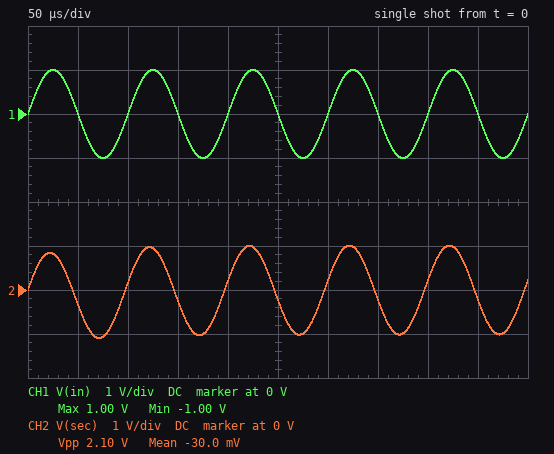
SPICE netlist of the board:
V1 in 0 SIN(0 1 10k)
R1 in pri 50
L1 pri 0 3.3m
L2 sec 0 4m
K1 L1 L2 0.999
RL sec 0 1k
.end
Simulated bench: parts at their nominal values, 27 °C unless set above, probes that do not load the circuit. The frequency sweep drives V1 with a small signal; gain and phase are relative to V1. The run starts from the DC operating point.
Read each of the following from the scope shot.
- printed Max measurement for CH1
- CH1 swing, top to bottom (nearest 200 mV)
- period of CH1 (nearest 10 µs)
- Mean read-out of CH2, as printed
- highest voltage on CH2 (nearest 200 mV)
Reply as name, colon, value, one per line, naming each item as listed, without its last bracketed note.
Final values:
printed Max measurement for CH1: 1.00 V
CH1 swing, top to bottom: 2.0 V
period of CH1: 100 µs
Mean read-out of CH2, as printed: -30.0 mV
highest voltage on CH2: 1.0 V
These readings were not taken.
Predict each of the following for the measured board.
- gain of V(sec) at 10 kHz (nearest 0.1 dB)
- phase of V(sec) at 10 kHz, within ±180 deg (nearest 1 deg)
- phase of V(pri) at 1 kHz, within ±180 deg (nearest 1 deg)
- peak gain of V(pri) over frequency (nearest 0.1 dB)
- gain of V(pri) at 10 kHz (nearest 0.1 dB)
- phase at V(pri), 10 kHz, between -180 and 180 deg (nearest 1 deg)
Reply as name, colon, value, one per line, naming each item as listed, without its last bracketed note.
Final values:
gain of V(sec) at 10 kHz: 0.1 dB
phase of V(sec) at 10 kHz, within ±180 deg: 13 deg
phase of V(pri) at 1 kHz, within ±180 deg: 66 deg
peak gain of V(pri) over frequency: 0 dB
gain of V(pri) at 10 kHz: -0.7 dB
phase at V(pri), 10 kHz, between -180 and 180 deg: 13 deg
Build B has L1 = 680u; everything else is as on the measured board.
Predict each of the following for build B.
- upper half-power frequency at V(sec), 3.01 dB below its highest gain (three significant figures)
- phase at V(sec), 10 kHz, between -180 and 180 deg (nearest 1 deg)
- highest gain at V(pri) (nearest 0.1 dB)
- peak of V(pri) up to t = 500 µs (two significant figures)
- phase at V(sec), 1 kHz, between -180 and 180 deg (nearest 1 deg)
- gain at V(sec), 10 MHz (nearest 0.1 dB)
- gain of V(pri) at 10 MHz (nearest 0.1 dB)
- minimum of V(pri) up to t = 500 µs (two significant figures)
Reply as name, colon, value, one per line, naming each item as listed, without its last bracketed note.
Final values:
upper half-power frequency at V(sec), 3.01 dB below its highest gain: 25.8 MHz
phase at V(sec), 10 kHz, between -180 and 180 deg: 42 deg
highest gain at V(pri): 0 dB
peak of V(pri) up to t = 500 µs: 570 mV
phase at V(sec), 1 kHz, between -180 and 180 deg: 84 deg
gain at V(sec), 10 MHz: 4.8 dB
gain of V(pri) at 10 MHz: -1.9 dB
minimum of V(pri) up to t = 500 µs: -580 mV
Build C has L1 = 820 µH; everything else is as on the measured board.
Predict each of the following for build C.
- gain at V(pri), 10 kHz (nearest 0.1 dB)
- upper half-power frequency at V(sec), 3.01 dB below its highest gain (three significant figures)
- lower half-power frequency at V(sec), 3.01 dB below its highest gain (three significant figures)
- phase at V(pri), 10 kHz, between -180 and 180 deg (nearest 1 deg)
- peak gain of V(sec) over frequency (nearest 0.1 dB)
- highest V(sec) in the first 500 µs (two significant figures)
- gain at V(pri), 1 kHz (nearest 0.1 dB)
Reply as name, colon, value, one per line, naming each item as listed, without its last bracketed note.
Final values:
gain at V(pri), 10 kHz: -4.0 dB
upper half-power frequency at V(sec), 3.01 dB below its highest gain: 24.8 MHz
lower half-power frequency at V(sec), 3.01 dB below its highest gain: 7.80 kHz
phase at V(pri), 10 kHz, between -180 and 180 deg: 38 deg
peak gain of V(sec) over frequency: 5.0 dB
highest V(sec) in the first 500 µs: 1.4 V
gain at V(pri), 1 kHz: -19.8 dB
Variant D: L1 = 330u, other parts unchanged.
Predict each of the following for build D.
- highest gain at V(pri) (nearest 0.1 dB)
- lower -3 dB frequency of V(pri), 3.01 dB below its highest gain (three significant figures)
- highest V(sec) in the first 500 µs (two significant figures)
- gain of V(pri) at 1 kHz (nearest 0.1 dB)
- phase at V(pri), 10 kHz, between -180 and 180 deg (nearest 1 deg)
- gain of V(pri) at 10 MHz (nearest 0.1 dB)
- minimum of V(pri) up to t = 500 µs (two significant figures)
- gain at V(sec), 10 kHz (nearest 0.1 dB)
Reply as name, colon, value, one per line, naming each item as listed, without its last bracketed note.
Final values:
highest gain at V(pri): 0 dB
lower -3 dB frequency of V(pri), 3.01 dB below its highest gain: 15.1 MHz
highest V(sec) in the first 500 µs: 1.2 V
gain of V(pri) at 1 kHz: -27.7 dB
phase at V(pri), 10 kHz, between -180 and 180 deg: 56 deg
gain of V(pri) at 10 MHz: -3.5 dB
minimum of V(pri) up to t = 500 µs: -350 mV
gain at V(sec), 10 kHz: 1.6 dB
